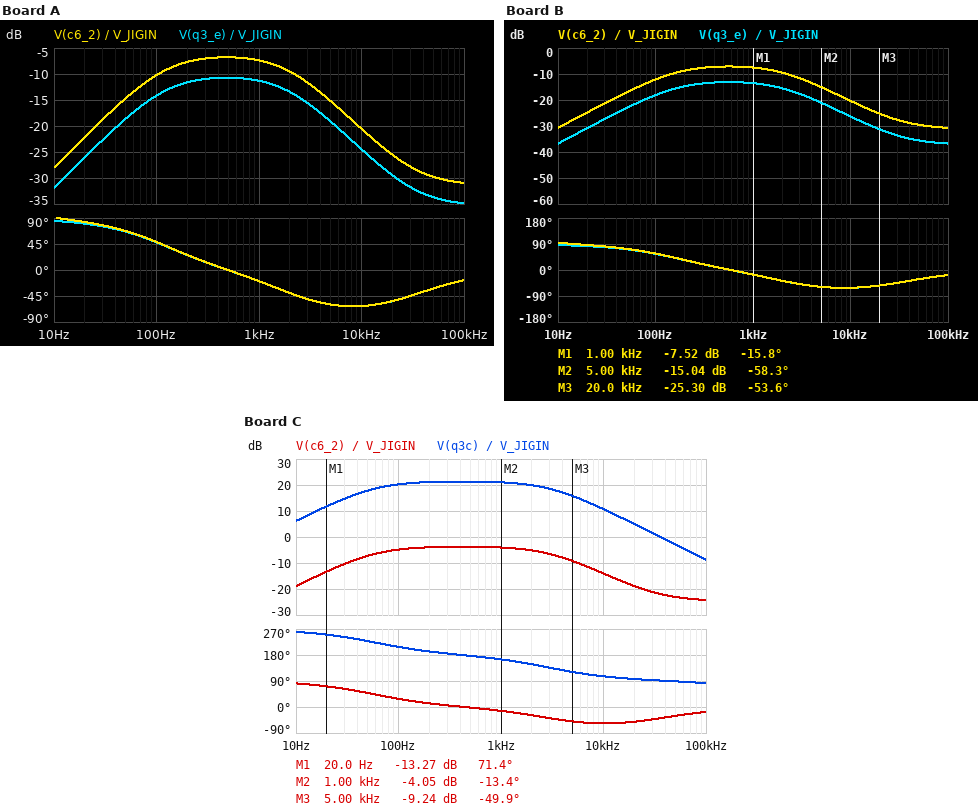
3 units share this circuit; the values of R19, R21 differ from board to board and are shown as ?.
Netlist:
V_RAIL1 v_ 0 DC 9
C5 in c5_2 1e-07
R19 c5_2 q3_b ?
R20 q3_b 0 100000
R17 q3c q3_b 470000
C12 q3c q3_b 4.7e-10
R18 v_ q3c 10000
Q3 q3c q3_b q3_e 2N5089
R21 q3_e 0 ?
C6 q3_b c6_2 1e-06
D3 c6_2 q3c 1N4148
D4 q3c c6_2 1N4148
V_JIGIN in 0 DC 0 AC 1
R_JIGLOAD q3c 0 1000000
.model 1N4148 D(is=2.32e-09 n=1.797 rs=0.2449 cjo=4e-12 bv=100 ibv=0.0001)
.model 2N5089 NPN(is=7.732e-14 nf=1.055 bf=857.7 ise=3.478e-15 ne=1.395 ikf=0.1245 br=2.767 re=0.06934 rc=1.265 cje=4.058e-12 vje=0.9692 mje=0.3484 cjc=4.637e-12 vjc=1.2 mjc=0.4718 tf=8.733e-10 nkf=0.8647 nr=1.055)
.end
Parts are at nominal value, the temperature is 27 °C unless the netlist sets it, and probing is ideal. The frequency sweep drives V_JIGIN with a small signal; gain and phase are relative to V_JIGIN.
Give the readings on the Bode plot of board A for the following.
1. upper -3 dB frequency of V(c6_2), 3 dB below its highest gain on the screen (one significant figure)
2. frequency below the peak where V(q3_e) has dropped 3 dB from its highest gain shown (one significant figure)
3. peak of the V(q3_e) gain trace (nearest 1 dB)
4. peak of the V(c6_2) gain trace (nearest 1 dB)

2 kHz
100 Hz
-11 dB
-7 dB
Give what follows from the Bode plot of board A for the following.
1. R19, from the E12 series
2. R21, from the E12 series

5.6 kΩ
100 Ω
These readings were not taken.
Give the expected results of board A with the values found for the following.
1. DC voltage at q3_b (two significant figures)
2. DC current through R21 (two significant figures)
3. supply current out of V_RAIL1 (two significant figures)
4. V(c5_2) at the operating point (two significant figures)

660 mV
480 µA
490 µA
660 mV
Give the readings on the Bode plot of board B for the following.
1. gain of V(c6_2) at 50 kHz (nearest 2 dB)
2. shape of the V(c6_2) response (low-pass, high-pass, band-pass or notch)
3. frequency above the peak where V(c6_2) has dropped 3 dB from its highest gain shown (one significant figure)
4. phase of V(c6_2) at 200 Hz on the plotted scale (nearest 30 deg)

-30 dB
band-pass
2 kHz
30 deg
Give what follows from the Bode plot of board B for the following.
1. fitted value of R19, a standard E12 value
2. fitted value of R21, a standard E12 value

3.9 kΩ
56 Ω
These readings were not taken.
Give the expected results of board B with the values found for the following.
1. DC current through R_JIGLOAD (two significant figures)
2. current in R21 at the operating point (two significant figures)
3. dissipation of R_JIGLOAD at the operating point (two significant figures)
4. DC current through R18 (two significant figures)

4.0 µA
490 µA
16 µW
500 µA
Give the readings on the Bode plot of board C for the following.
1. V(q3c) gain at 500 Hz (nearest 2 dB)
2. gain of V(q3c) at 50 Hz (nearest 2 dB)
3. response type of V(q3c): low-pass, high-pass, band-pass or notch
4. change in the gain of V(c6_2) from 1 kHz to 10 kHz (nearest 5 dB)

22 dB
18 dB
band-pass
-10 dB
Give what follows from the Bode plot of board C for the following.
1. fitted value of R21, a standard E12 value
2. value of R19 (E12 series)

470 Ω
8.2 kΩ
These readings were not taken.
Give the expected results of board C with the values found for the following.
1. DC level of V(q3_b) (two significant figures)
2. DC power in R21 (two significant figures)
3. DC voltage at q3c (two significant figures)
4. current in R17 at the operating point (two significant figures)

800 mV
77 µW
4.8 V
8.6 µA
